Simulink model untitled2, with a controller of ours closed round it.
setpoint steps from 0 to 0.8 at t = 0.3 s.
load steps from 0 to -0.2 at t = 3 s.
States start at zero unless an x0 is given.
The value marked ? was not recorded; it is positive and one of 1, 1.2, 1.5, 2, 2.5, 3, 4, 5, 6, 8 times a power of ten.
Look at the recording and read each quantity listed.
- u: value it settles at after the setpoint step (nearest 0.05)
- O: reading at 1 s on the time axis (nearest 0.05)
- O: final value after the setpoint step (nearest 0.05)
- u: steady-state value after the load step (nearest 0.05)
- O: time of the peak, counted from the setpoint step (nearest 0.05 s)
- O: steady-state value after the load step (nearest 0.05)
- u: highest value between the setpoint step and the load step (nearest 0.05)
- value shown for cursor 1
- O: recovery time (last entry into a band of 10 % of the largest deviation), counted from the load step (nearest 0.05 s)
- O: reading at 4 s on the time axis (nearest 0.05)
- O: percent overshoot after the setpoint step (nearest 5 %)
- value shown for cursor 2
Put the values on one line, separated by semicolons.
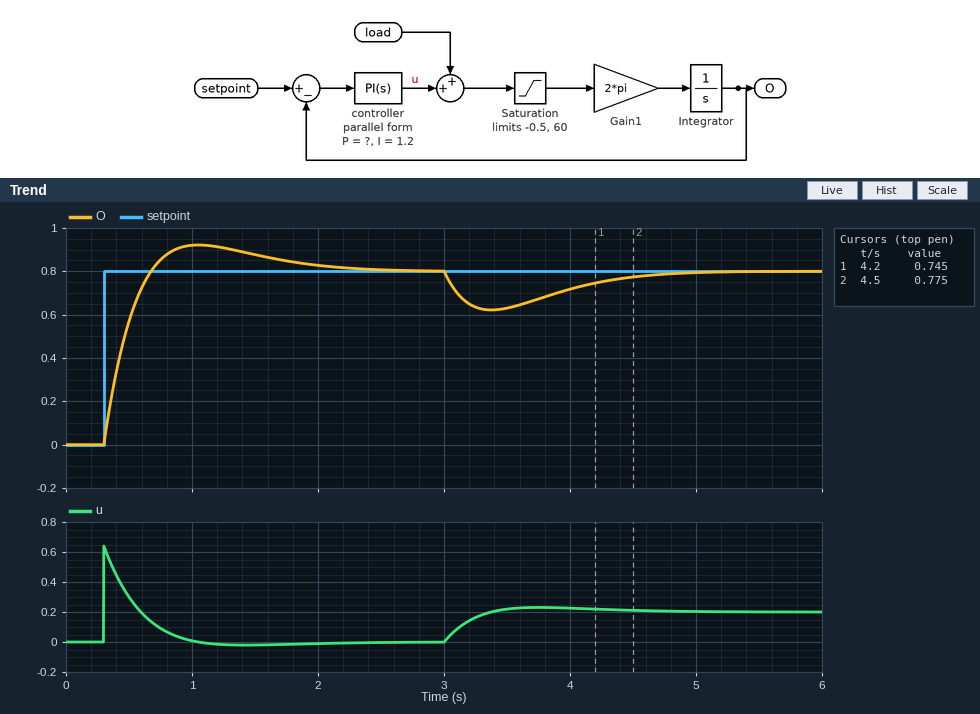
0.00; 0.90; 0.80; 0.20; 0.75 s; 0.80; 0.65; 0.745; 1.65 s; 0.70; 15 %; 0.775
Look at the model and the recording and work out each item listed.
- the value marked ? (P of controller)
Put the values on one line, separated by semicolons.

0.8
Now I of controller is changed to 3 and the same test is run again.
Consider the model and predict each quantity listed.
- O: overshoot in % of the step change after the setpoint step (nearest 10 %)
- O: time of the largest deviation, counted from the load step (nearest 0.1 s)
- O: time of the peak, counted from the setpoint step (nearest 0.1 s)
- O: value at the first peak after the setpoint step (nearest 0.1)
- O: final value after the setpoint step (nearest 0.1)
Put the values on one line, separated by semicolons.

30 %; 0.3 s; 0.5 s; 1.0; 0.8
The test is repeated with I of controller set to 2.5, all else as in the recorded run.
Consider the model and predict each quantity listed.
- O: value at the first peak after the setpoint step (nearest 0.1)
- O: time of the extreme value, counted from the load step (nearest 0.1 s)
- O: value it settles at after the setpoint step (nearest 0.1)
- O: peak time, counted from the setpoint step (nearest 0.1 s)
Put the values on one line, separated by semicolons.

1.0; 0.3 s; 0.8; 0.6 s
